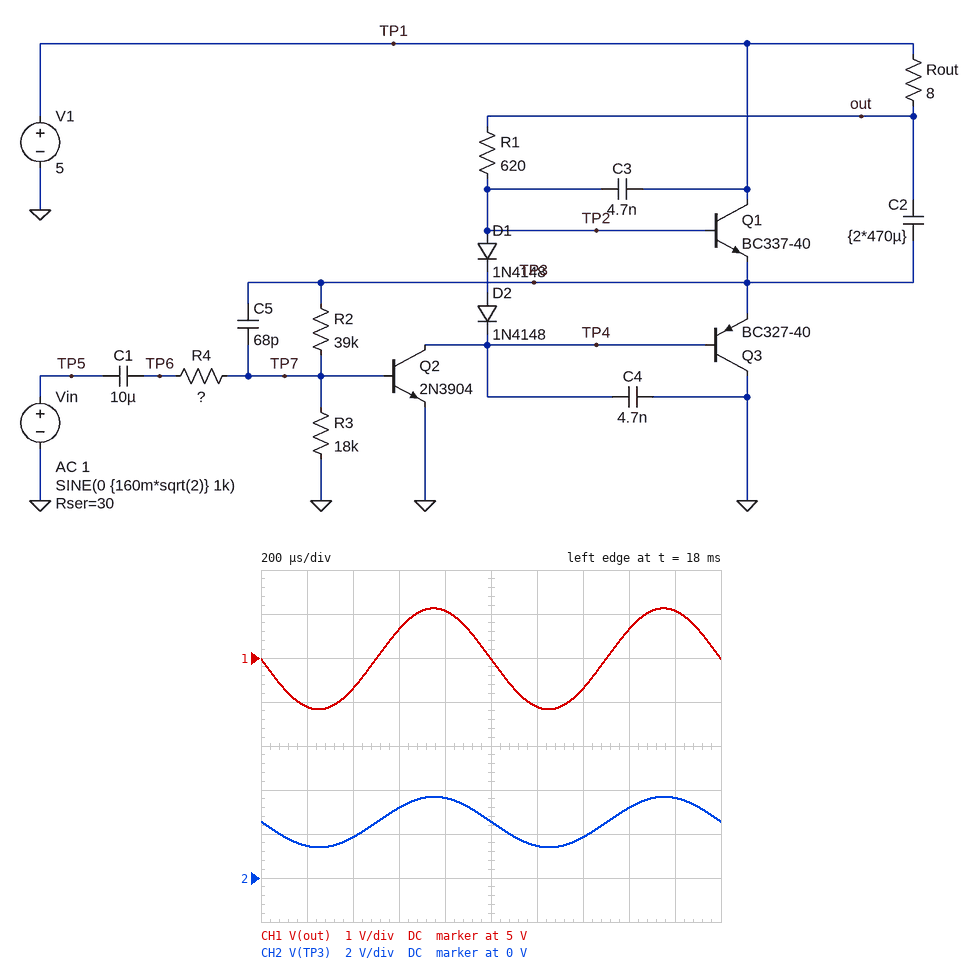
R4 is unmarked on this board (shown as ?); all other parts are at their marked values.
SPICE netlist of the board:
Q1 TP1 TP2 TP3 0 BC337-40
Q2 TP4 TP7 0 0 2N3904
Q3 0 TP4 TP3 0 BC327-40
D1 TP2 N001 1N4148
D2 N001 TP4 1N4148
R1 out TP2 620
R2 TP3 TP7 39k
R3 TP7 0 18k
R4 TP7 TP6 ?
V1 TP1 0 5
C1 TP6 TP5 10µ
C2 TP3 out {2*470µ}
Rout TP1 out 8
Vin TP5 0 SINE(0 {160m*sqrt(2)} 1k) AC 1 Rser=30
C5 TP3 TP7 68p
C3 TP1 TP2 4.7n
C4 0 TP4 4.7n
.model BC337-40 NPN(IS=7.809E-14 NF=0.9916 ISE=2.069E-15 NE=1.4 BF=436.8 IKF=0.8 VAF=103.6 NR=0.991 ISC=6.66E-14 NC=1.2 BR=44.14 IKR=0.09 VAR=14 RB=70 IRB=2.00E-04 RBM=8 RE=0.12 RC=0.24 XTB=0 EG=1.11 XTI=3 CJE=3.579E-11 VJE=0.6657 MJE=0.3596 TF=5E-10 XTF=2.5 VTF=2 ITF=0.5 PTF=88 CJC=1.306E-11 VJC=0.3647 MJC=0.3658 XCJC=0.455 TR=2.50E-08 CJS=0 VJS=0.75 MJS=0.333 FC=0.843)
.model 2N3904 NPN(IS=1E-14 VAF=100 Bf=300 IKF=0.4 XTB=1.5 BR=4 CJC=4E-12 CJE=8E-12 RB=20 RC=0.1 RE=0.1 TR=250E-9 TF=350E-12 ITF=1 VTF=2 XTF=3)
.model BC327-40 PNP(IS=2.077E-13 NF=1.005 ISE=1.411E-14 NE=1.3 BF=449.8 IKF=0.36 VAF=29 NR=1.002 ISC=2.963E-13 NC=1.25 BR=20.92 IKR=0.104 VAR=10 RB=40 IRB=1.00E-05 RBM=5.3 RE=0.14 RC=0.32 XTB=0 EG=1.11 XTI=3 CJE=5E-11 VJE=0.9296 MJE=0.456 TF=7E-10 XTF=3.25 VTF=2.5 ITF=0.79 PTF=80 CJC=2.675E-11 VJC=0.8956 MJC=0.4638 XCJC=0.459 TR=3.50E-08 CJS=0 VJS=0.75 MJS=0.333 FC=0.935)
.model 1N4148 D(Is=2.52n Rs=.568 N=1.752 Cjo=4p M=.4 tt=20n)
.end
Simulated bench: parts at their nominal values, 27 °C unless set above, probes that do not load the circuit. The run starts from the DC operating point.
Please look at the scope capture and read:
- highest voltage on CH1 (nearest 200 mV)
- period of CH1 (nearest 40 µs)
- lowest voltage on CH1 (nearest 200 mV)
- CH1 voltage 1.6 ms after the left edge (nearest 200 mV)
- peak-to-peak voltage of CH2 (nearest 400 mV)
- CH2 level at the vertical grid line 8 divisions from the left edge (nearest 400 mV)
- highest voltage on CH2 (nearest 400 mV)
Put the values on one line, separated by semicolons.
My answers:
6.2 V; 1.00 ms; 3.8 V; 5.6 V; 2.4 V; 3.2 V; 3.6 V
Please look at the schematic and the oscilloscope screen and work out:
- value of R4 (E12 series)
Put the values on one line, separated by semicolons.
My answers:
6.8 kΩ
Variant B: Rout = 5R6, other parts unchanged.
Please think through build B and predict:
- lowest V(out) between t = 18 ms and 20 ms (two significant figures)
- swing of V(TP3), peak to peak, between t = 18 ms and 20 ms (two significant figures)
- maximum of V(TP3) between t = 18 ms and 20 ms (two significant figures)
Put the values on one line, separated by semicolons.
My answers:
3.9 V; 2.2 V; 3.6 V
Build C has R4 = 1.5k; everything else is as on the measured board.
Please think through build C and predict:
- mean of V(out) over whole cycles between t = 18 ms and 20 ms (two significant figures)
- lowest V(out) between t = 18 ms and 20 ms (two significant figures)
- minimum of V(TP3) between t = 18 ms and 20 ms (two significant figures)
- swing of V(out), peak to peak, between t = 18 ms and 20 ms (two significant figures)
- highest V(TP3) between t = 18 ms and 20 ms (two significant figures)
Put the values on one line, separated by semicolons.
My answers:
5.0 V; 3.0 V; 850 mV; 4.0 V; 4.8 V
